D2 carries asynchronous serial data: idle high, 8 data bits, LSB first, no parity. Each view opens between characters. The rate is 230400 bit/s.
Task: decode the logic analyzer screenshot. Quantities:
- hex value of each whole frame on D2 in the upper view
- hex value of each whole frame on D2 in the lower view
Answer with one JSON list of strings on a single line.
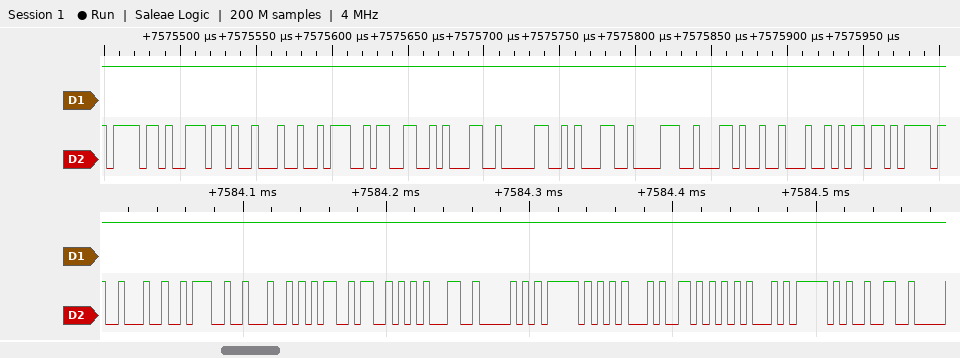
["6F, 6E, 22, 3A, 33, 31, 30, 31, 38, 2C, 22, 6D", "22, 3A, 22, 35, 53, 31, 50, 5F, 45, 56, 45, 5F, 32"]
